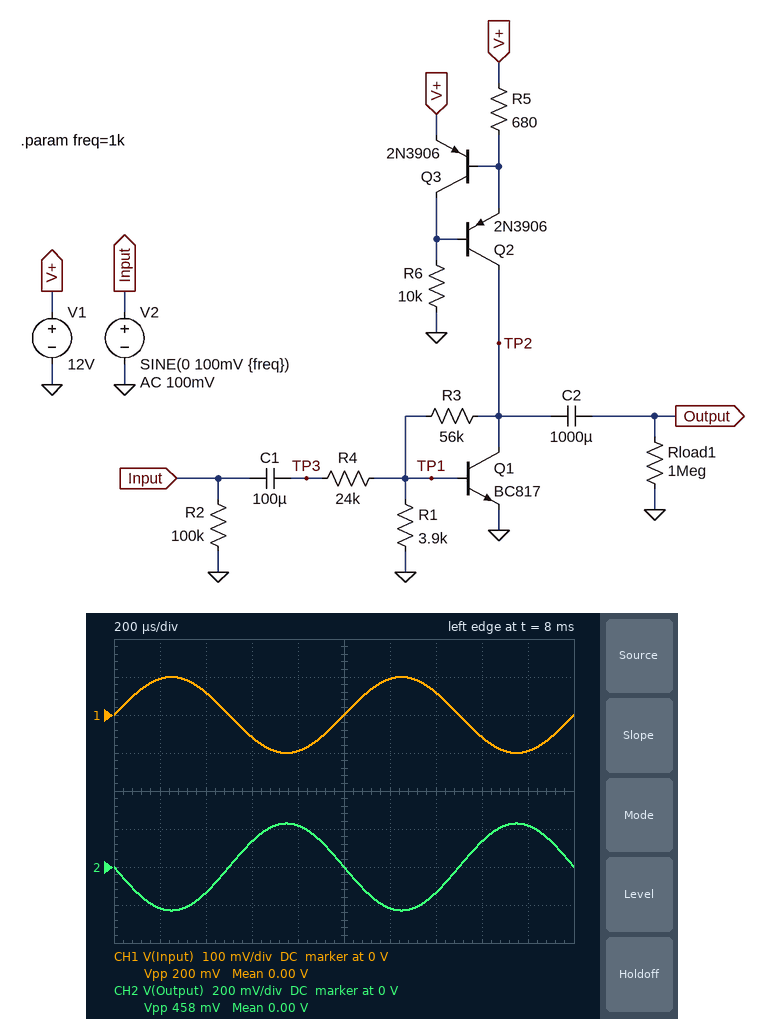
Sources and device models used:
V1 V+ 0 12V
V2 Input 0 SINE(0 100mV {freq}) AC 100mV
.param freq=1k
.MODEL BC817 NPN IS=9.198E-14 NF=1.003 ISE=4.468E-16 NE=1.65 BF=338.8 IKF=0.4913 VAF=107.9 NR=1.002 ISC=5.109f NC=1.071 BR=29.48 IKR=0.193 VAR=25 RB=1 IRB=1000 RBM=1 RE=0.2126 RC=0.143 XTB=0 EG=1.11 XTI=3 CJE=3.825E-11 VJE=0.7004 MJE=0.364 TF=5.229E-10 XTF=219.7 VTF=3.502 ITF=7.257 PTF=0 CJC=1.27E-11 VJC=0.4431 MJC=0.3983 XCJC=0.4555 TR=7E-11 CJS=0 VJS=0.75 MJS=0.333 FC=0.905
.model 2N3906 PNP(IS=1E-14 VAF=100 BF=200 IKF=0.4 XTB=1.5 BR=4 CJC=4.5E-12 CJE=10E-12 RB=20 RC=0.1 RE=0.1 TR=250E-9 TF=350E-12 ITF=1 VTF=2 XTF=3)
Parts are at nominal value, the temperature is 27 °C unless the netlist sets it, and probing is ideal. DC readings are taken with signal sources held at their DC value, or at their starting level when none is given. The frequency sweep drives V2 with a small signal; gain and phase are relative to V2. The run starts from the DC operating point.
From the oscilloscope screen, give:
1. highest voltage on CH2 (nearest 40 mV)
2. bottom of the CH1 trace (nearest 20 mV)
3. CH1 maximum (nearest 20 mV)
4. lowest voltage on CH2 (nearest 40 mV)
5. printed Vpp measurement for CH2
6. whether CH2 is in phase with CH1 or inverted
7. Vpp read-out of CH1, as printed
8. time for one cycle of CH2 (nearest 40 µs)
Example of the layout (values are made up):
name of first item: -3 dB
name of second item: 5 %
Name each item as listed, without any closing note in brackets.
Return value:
highest voltage on CH2: 240 mV
bottom of the CH1 trace: -100 mV
CH1 maximum: 100 mV
lowest voltage on CH2: -240 mV
printed Vpp measurement for CH2: 458 mV
whether CH2 is in phase with CH1 or inverted: inverted
Vpp read-out of CH1, as printed: 200 mV
time for one cycle of CH2: 1.00 ms
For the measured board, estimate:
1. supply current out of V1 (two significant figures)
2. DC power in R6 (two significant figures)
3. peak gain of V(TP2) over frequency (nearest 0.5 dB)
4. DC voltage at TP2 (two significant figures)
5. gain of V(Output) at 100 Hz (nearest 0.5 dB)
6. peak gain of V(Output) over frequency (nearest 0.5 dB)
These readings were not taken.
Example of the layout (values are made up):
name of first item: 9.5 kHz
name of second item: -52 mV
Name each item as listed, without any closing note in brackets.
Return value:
supply current out of V1: 2.0 mA
DC power in R6: 11 mW
peak gain of V(TP2) over frequency: 7.0 dB
DC voltage at TP2: 9.2 V
gain of V(Output) at 100 Hz: 7.0 dB
peak gain of V(Output) over frequency: 7.0 dB
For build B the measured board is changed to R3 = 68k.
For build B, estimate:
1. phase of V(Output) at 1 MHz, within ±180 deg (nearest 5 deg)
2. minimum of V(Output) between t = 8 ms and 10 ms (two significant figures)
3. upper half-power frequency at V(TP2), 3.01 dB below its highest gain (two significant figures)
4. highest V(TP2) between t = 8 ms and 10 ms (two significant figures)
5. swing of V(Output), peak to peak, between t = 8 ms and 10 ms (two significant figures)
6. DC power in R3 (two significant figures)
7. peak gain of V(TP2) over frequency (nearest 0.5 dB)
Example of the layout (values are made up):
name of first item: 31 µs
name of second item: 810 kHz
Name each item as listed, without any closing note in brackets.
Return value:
phase of V(Output) at 1 MHz, within ±180 deg: 120 deg
minimum of V(Output) between t = 8 ms and 10 ms: -280 mV
upper half-power frequency at V(TP2), 3.01 dB below its highest gain: 660 kHz
highest V(TP2) between t = 8 ms and 10 ms: 11 V
swing of V(Output), peak to peak, between t = 8 ms and 10 ms: 500 mV
DC power in R3: 1.6 mW
peak gain of V(TP2) over frequency: 9.0 dB
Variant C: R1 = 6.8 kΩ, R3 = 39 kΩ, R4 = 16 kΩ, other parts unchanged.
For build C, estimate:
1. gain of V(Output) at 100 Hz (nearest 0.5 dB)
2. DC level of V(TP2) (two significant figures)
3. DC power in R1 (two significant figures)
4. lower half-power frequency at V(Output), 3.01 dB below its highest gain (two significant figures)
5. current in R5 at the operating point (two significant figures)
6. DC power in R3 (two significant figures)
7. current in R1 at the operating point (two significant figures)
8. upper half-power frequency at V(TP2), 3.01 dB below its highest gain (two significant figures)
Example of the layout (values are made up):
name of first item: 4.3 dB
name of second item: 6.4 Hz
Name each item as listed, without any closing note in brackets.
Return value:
gain of V(Output) at 100 Hz: 7.5 dB
DC level of V(TP2): 4.1 V
DC power in R1: 52 µW
lower half-power frequency at V(Output), 3.01 dB below its highest gain: 99 mHz
current in R5 at the operating point: 970 µA
DC power in R3: 320 µW
current in R1 at the operating point: 88 µA
upper half-power frequency at V(TP2), 3.01 dB below its highest gain: 770 kHz
